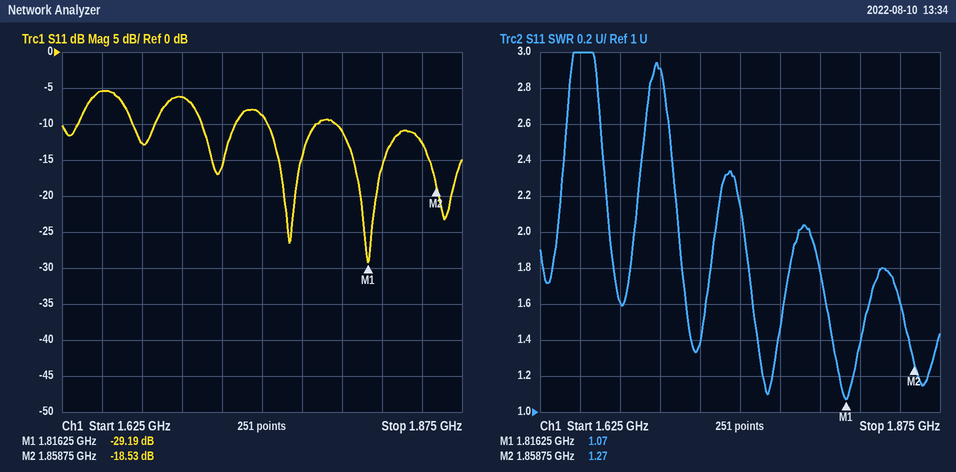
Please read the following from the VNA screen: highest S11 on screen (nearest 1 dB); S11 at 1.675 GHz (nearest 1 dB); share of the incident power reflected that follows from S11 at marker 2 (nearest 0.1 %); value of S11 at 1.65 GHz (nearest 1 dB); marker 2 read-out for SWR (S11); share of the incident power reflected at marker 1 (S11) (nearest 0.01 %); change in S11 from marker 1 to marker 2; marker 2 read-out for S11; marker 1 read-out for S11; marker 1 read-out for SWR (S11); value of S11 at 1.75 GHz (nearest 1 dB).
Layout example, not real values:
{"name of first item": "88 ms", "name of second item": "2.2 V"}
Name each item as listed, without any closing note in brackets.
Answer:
{"highest S11 on screen": "-5 dB", "S11 at 1.675 GHz": "-13 dB", "share of the incident power reflected that follows from S11 at marker 2": "1.4 %", "value of S11 at 1.65 GHz": "-5 dB", "marker 2 read-out for SWR": "1.27", "share of the incident power reflected at marker 1 (S11)": "0.12 %", "change in S11 from marker 1 to marker 2": "10.66 dB", "marker 2 read-out for S11": "-18.53 dB", "marker 1 read-out for S11": "-29.19 dB", "marker 1 read-out for SWR": "1.07", "value of S11 at 1.75 GHz": "-9 dB"}
